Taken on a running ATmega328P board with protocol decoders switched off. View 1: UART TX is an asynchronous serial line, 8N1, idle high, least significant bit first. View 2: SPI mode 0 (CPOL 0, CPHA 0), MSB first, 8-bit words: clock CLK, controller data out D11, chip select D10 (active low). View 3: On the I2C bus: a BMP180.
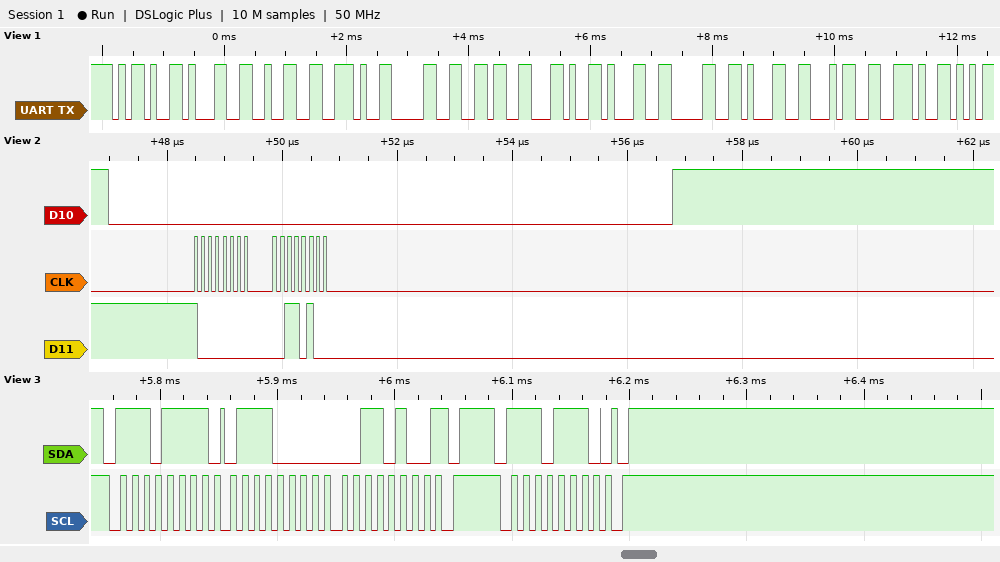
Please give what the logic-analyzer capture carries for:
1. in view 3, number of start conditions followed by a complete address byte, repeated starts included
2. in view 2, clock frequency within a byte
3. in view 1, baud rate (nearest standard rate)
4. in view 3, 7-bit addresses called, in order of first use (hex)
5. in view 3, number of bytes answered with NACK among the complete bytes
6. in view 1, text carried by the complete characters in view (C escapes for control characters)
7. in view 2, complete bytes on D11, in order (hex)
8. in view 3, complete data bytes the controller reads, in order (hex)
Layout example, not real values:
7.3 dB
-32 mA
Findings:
2
8 MHz
9600 baud
0x77
1
"-12.06,1014."
80 34
70 34
